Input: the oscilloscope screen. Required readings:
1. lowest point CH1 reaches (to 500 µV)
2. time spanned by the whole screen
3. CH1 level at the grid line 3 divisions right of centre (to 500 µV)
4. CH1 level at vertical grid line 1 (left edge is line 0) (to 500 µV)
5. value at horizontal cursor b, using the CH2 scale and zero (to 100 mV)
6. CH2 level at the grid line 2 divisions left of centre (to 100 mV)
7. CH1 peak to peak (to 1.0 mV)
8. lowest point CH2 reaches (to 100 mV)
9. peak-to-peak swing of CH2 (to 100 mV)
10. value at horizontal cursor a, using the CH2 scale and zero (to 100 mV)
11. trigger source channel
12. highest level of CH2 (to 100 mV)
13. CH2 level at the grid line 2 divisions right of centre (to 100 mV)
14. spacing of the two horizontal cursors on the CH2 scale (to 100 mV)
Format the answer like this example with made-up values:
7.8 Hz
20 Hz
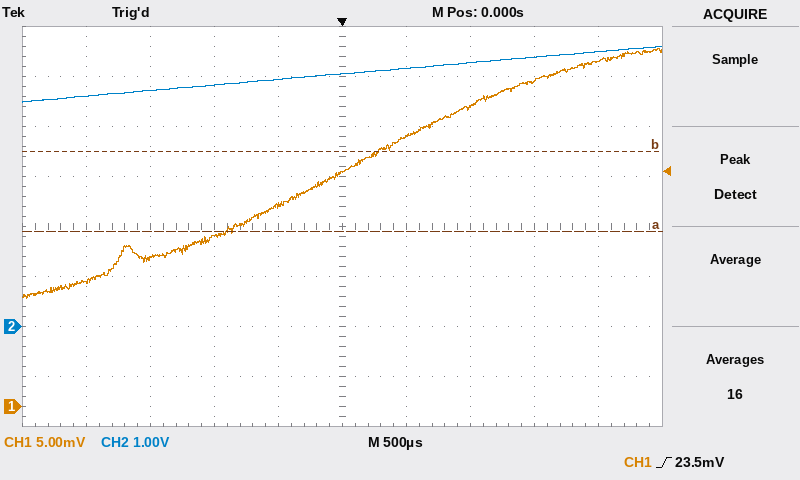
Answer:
11.0 mV
5 ms
32.5 mV
12.5 mV
3.5 V
4.8 V
25.0 mV
4.5 V
1.1 V
1.9 V
CH1
5.6 V
5.3 V
1.6 V
